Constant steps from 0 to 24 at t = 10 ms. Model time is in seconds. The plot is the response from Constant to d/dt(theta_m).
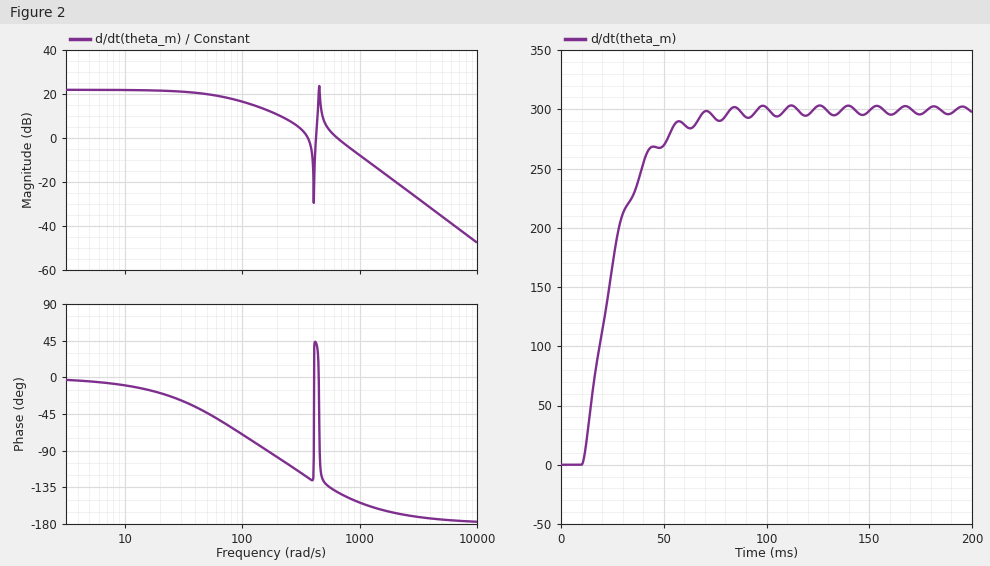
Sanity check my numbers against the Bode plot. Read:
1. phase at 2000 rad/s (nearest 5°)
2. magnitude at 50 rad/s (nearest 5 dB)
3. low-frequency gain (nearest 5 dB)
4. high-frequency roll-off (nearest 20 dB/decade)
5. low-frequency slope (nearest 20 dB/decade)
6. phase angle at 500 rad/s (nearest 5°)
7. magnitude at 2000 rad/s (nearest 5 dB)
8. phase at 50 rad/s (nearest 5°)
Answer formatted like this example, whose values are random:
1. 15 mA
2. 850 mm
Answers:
1. -165°
2. 20 dB
3. 20 dB
4. -40 dB/decade
5. 0 dB/decade
6. -130°
7. -20 dB
8. -45°
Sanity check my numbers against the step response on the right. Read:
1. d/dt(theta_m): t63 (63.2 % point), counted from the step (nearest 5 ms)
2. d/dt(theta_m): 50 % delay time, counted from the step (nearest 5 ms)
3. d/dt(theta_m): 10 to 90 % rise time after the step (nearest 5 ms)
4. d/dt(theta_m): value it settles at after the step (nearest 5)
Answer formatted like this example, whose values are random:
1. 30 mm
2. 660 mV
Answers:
1. 15 ms
2. 15 ms
3. 35 ms
4. 300
